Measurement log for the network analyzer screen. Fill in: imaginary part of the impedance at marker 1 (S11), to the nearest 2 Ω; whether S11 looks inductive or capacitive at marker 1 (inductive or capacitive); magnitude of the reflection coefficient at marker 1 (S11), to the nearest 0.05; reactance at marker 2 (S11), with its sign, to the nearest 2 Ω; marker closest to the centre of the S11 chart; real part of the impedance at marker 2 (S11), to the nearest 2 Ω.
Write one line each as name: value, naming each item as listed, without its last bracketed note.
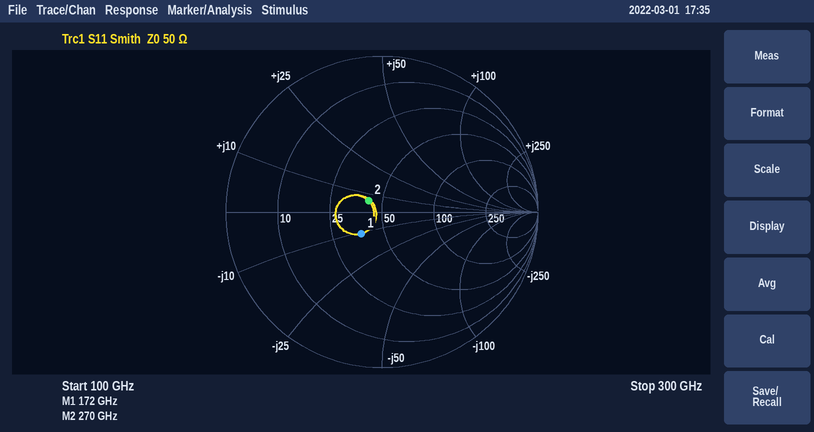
imaginary part of the impedance at marker 1 (S11), to the nearest 2 Ω: -10 Ω
whether S11 looks inductive or capacitive at marker 1: capacitive
magnitude of the reflection coefficient at marker 1 (S11), to the nearest 0.05: 0.20
reactance at marker 2 (S11), with its sign, to the nearest 2 Ω: +6 Ω
marker closest to the centre of the S11 chart: marker 2
real part of the impedance at marker 2 (S11), to the nearest 2 Ω: 42 Ω
